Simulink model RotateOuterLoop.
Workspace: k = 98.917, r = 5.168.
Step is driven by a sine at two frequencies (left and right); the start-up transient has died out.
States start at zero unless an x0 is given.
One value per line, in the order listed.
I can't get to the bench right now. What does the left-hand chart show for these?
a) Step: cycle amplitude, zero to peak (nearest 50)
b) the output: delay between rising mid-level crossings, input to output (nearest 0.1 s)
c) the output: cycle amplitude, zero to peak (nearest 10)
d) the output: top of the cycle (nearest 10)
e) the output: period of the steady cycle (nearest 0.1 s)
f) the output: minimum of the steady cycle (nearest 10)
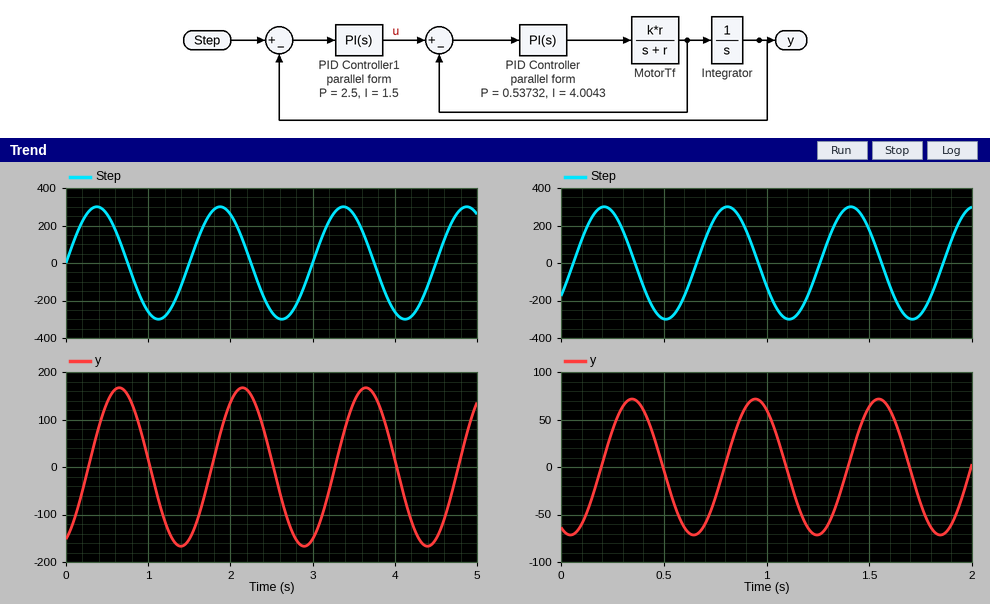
300
0.3 s
170
170
1.5 s
-170
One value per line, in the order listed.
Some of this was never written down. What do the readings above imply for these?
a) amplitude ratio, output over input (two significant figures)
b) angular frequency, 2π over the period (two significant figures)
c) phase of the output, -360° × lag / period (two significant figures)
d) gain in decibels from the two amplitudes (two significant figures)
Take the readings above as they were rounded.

0.57
4.2 rad/s
-72°
-4.9 dB
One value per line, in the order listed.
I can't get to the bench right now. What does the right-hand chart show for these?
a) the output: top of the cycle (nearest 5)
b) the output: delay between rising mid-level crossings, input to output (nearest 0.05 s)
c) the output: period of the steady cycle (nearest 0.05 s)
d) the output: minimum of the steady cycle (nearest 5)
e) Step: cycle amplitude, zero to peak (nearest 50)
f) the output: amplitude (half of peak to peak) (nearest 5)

70
0.15 s
0.60 s
-70
300
70
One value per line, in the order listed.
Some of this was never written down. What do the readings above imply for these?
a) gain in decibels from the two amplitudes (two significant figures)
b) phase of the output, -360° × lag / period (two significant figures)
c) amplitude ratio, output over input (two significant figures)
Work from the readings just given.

-13 dB
-90°
0.23
